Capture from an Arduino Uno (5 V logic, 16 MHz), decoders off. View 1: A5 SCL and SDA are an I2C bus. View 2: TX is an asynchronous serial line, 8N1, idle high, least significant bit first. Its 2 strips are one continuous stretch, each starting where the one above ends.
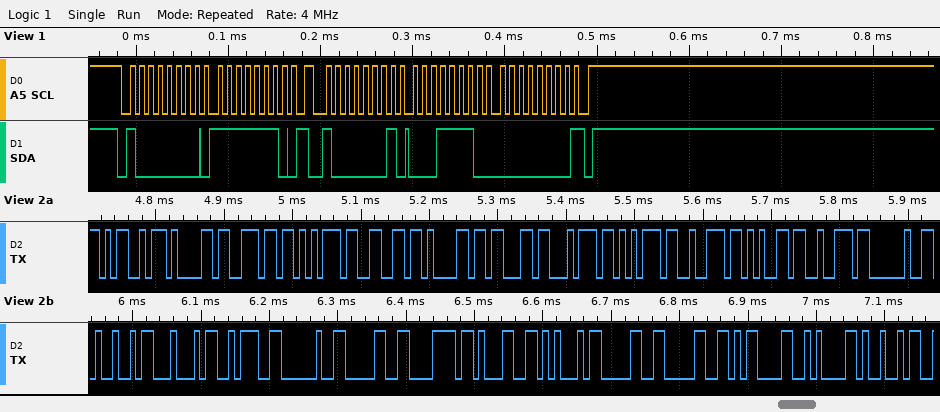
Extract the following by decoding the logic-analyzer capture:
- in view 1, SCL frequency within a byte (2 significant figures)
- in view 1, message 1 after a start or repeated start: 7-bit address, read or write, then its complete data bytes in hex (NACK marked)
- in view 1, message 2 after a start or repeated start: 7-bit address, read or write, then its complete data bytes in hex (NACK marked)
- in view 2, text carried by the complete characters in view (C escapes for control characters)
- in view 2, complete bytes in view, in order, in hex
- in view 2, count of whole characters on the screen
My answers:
100 kHz
0x40 write: FE
0x40 read: 1E 00 NACK
"Manufacturer ID: 0x1E00\r\nI"
4D 61 6E 75 66 61 63 74 75 72 65 72 20 49 44 3A 20 30 78 31 45 30 30 0D 0A 49
26
